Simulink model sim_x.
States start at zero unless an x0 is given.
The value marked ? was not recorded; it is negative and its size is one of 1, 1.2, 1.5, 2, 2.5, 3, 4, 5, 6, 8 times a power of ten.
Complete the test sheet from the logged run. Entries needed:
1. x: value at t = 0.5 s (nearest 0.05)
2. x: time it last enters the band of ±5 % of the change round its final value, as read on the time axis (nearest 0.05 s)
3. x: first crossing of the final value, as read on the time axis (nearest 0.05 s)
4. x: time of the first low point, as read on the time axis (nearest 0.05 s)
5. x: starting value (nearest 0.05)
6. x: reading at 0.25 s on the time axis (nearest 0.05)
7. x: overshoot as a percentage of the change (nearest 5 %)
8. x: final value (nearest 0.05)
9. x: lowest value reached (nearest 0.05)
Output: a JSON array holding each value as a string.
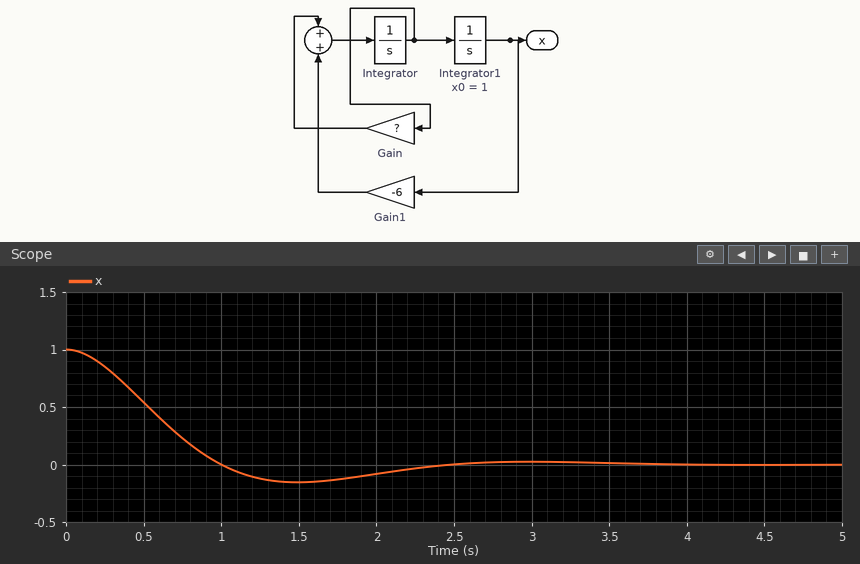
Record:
["0.55", "2.15 s", "1.00 s", "1.50 s", "1.00", "0.85", "15 %", "0.00", "-0.15"]
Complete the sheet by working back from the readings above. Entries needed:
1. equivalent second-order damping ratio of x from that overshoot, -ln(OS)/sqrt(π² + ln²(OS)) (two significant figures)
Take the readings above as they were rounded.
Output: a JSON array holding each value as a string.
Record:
["0.52"]
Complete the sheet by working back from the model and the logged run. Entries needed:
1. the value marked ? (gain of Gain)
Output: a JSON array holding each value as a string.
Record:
["-2.5"]
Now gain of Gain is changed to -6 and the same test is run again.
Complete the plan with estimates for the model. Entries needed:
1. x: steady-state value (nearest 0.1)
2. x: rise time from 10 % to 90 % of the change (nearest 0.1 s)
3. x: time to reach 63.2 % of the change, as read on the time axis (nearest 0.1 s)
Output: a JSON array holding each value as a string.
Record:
["0.0", "1.8 s", "1.0 s"]
